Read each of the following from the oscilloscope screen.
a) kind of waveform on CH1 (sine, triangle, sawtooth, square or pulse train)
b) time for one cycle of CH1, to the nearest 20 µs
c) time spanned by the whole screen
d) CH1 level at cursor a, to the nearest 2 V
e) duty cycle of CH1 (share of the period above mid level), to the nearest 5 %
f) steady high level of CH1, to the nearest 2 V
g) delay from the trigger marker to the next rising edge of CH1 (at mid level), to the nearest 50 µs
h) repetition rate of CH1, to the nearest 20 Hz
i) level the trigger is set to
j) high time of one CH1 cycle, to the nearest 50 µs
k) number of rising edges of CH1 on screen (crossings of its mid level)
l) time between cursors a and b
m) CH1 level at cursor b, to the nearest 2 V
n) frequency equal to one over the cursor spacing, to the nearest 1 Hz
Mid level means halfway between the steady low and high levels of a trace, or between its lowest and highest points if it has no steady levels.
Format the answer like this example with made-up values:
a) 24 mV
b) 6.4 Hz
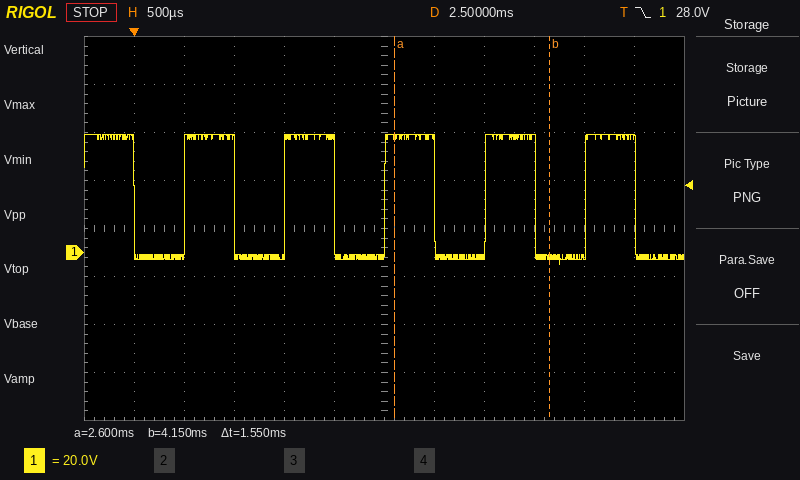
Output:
a) square
b) 1.00 ms
c) 6 ms
d) 48 V
e) 50 %
f) 48 V
g) 500 µs
h) 1.00 kHz
i) 28.0 V
j) 500 µs
k) 5
l) 1.55 ms
m) -2 V
n) 645 Hz
